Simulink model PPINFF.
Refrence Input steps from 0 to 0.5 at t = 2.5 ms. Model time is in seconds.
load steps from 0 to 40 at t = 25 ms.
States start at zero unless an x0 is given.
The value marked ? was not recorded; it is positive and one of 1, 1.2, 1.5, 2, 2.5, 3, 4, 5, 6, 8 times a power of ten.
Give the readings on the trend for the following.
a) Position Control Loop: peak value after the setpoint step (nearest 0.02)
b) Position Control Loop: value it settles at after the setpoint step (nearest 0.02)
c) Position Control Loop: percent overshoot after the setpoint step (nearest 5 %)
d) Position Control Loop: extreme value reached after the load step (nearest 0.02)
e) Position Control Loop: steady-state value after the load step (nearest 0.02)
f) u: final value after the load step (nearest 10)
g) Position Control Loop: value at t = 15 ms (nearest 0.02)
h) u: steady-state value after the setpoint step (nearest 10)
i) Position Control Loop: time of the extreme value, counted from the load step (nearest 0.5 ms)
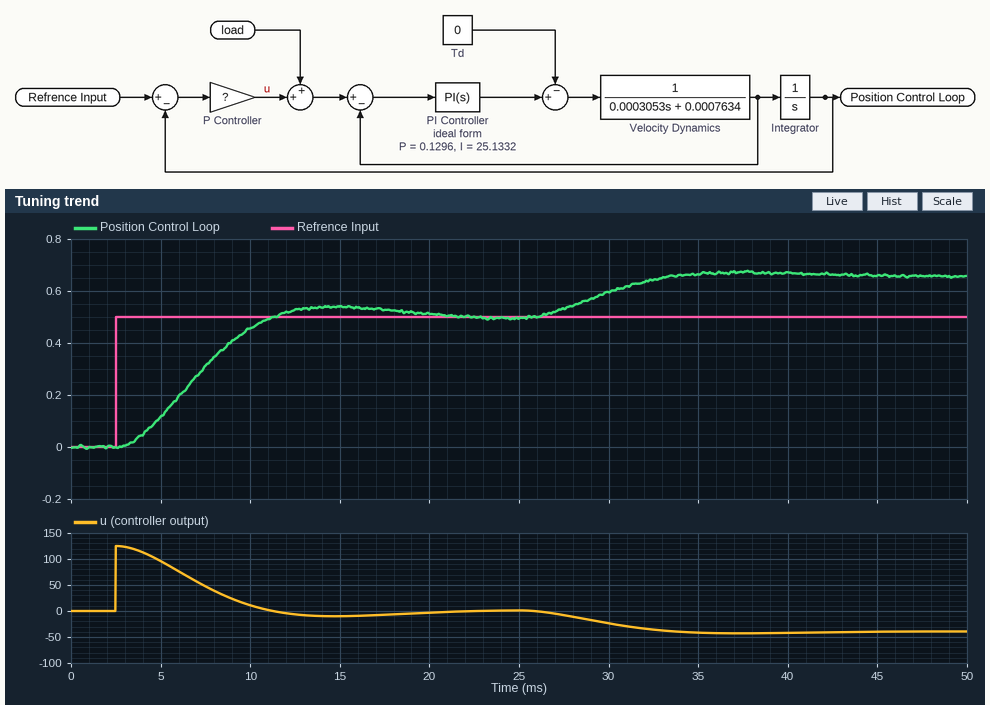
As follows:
0.54
0.50
10 %
0.68
0.66
-40
0.54
0
12.5 ms
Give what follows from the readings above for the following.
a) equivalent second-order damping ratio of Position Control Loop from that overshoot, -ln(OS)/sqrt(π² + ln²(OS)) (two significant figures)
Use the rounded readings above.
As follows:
0.59
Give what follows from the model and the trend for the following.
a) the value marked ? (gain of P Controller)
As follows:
250
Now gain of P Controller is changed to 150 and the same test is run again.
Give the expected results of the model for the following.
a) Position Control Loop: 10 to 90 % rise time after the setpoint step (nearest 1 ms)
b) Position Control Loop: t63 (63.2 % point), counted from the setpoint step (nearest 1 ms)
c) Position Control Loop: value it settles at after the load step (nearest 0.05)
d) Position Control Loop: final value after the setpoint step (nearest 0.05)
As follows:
10 ms
7 ms
0.75
0.50
